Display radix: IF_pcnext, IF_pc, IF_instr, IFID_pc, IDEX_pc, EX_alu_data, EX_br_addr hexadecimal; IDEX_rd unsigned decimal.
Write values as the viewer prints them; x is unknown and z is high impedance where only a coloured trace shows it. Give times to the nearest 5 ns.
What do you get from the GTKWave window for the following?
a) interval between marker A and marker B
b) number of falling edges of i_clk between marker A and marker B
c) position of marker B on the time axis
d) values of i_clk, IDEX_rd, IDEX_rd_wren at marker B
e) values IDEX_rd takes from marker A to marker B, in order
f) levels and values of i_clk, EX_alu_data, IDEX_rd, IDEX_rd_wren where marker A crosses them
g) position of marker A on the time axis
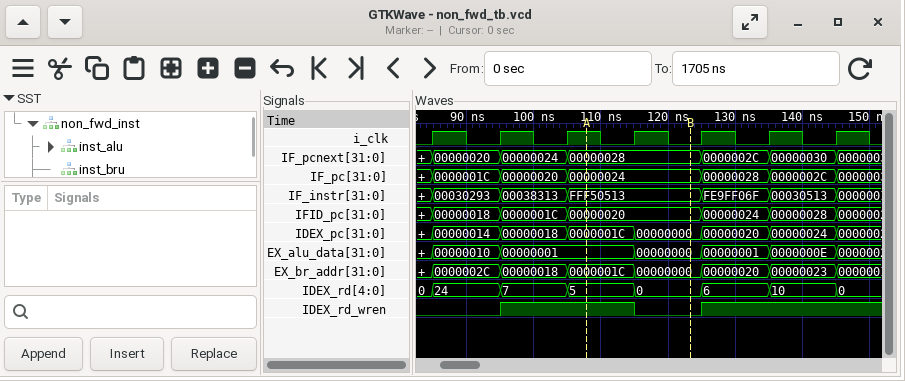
15 ns
2
125 ns
i_clk=0, IDEX_rd=0, IDEX_rd_wren=0
5, 0
i_clk=1, EX_alu_data=00000001, IDEX_rd=5, IDEX_rd_wren=1
110 ns
